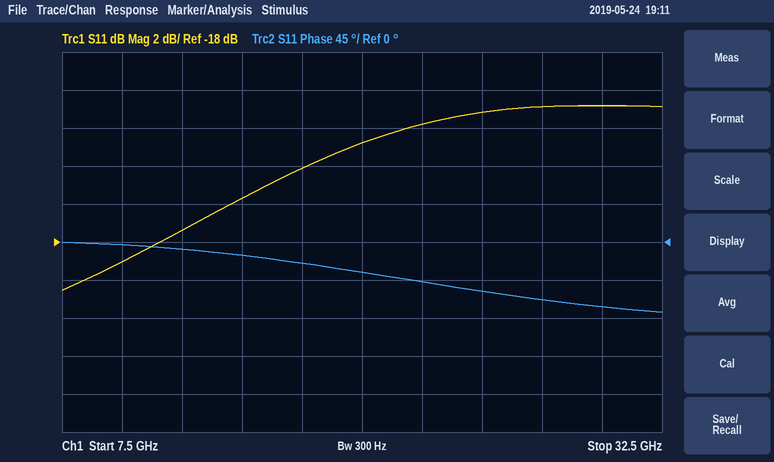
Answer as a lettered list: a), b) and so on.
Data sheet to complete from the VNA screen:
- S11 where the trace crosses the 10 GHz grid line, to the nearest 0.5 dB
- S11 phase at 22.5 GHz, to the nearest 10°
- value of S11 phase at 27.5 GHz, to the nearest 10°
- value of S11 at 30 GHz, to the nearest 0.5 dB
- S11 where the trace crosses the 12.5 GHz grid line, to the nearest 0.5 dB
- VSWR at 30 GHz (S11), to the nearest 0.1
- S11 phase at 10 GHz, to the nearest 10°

a) -19.0 dB
b) -50°
c) -70°
d) -11.0 dB
e) -17.5 dB
f) 1.8
g) 0°
